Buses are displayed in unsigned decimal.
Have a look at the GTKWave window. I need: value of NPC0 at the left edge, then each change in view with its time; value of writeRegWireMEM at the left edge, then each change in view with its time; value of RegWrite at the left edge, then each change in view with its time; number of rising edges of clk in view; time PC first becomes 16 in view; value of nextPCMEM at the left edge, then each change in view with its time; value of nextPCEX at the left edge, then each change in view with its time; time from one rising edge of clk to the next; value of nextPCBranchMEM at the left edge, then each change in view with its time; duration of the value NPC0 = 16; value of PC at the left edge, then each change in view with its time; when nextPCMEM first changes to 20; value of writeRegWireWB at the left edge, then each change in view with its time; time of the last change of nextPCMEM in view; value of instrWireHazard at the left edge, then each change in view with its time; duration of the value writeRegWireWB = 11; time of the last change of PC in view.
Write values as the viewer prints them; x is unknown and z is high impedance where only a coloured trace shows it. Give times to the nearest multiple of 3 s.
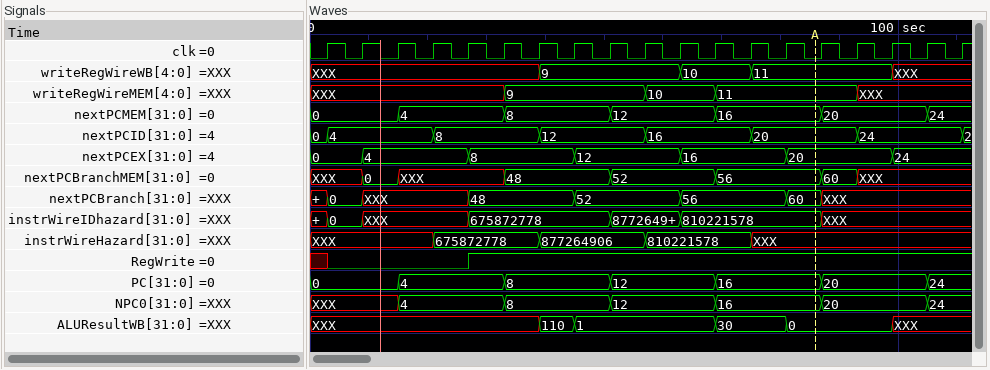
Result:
XXX, 4 at 15 s, 8 at 33 s, 12 at 51 s, 16 at 69 s, 20 at 87 s, 24 at 105 s
XXX, 9 at 33 s, 10 at 57 s, 11 at 69 s, XXX at 93 s
x, 0 at 3 s, 1 at 27 s
19
69 s
0, 4 at 15 s, 8 at 33 s, 12 at 51 s, 16 at 69 s, 20 at 87 s, 24 at 105 s
0, 4 at 9 s, 8 at 27 s, 12 at 45 s, 16 at 63 s, 20 at 81 s, 24 at 99 s
6 s
XXX, 0 at 9 s, XXX at 15 s, 48 at 33 s, 52 at 51 s, 56 at 69 s, 60 at 87 s, XXX at 93 s
18 s
0, 4 at 15 s, 8 at 33 s, 12 at 51 s, 16 at 69 s, 20 at 87 s, 24 at 105 s
87 s
XXX, 9 at 39 s, 10 at 63 s, 11 at 75 s, XXX at 99 s
105 s
XXX, 675872778 at 21 s, 877264906 at 39 s, 810221578 at 57 s, XXX at 75 s
24 s
105 s
